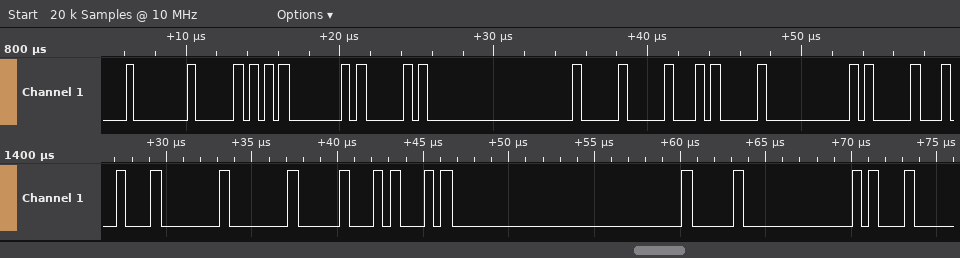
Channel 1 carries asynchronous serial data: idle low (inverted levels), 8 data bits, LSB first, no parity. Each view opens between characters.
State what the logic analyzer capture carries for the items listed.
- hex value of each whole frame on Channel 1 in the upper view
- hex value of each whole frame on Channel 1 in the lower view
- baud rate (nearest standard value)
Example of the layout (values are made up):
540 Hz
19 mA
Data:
7F, D5, 7D, FF, DF, D7, FF, 7D
F7, 7F, D7, FD, DF, DD
2000000 baud
